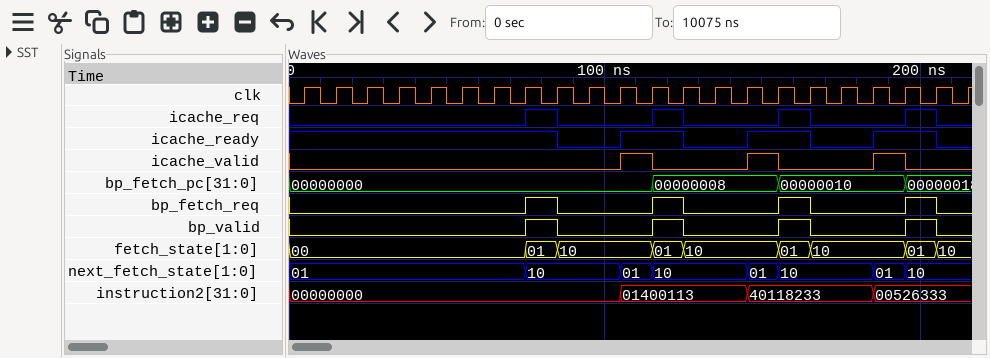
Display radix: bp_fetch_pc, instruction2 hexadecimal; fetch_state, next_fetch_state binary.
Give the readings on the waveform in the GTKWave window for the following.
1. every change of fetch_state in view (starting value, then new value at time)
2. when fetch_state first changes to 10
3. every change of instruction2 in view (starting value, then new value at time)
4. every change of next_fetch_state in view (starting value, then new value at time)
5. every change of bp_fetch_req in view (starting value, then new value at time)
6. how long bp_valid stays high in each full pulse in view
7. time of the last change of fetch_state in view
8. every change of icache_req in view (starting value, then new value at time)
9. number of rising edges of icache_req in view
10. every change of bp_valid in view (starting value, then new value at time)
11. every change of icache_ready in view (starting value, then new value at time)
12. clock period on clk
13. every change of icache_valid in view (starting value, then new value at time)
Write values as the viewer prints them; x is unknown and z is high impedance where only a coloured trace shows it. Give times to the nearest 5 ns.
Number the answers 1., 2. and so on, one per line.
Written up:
1. 00, 01 at 75 ns, 10 at 85 ns, 01 at 115 ns, 10 at 125 ns, 01 at 155 ns, 10 at 165 ns, 01 at 195 ns, 10 at 205 ns
2. 85 ns
3. 00000000, 01400113 at 105 ns, 40118233 at 145 ns, 00526333 at 185 ns
4. 01, 10 at 75 ns, 01 at 105 ns, 10 at 115 ns, 01 at 145 ns, 10 at 155 ns, 01 at 185 ns, 10 at 195 ns
5. 0, 1 at 75 ns, 0 at 85 ns, 1 at 115 ns, 0 at 125 ns, 1 at 155 ns, 0 at 165 ns, 1 at 195 ns, 0 at 205 ns
6. 10 ns, 10 ns, 10 ns, 10 ns
7. 205 ns
8. 0, 1 at 75 ns, 0 at 85 ns, 1 at 115 ns, 0 at 125 ns, 1 at 155 ns, 0 at 165 ns, 1 at 195 ns, 0 at 205 ns
9. 4
10. 0, 1 at 75 ns, 0 at 85 ns, 1 at 115 ns, 0 at 125 ns, 1 at 155 ns, 0 at 165 ns, 1 at 195 ns, 0 at 205 ns
11. 1, 0 at 85 ns, 1 at 105 ns, 0 at 125 ns, 1 at 145 ns, 0 at 165 ns, 1 at 185 ns, 0 at 205 ns
12. 10 ns
13. 0, 1 at 105 ns, 0 at 115 ns, 1 at 145 ns, 0 at 155 ns, 1 at 185 ns, 0 at 195 ns
